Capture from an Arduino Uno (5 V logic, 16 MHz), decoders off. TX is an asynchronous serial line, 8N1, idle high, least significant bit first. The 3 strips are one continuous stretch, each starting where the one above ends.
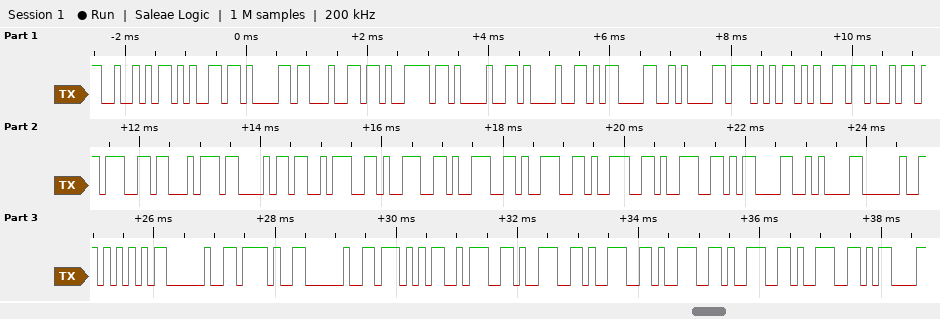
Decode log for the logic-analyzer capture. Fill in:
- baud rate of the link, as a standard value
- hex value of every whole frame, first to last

9600 baud
52 65 61 64 79 21 21 0D 0A 57 65 69 67 74 68 3A 39 39 39 39 39 0D 0A 20 55 20 2F 20 57 3A 39 39 39 39 39 0D
